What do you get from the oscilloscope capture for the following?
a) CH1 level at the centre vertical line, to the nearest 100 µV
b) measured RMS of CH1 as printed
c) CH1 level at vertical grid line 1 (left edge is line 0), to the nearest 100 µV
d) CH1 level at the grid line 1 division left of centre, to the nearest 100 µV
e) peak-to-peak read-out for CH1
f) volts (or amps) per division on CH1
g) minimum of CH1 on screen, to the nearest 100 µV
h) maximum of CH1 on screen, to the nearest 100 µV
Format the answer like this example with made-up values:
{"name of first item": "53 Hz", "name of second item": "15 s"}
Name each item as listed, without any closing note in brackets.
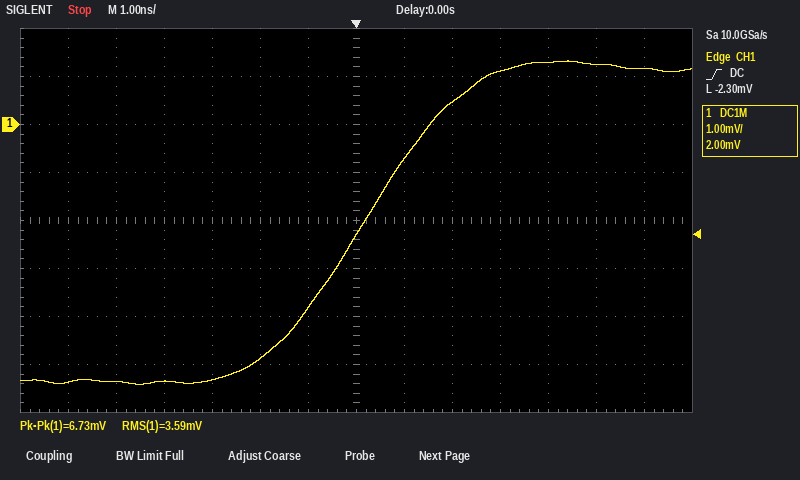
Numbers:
{"CH1 level at the centre vertical line, to the nearest 100 µV": "-2.3 mV", "measured RMS of CH1 as printed": "3.59 mV", "CH1 level at vertical grid line 1 (left edge is line 0), to the nearest 100 µV": "-5.4 mV", "CH1 level at the grid line 1 division left of centre, to the nearest 100 µV": "-3.8 mV", "peak-to-peak read-out for CH1": "6.73 mV", "volts (or amps) per division on CH1": "1 mV", "minimum of CH1 on screen, to the nearest 100 µV": "-5.4 mV", "maximum of CH1 on screen, to the nearest 100 µV": "1.3 mV"}
